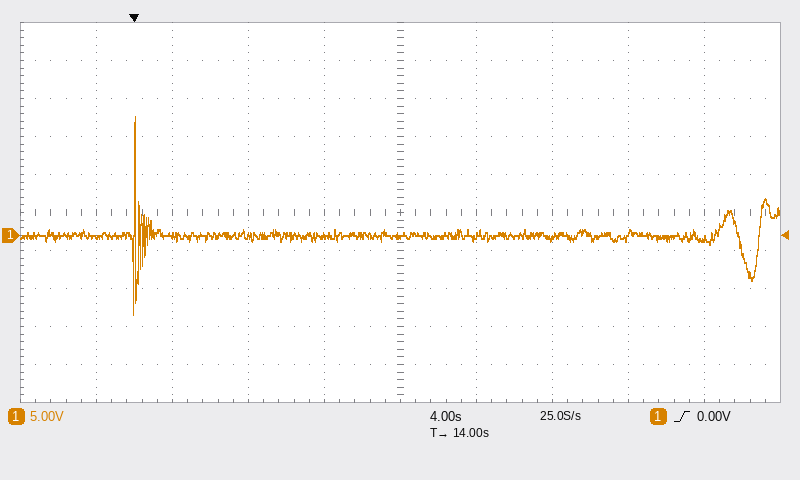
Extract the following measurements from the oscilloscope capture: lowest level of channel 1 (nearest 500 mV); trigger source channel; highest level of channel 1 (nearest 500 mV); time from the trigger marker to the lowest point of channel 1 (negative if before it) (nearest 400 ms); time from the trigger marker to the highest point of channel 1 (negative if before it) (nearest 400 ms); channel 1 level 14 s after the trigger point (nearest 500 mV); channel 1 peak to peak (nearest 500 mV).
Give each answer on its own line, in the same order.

-10.5 V
channel 1
15.5 V
0.0 s
0.0 s
0.0 V
26.0 V
